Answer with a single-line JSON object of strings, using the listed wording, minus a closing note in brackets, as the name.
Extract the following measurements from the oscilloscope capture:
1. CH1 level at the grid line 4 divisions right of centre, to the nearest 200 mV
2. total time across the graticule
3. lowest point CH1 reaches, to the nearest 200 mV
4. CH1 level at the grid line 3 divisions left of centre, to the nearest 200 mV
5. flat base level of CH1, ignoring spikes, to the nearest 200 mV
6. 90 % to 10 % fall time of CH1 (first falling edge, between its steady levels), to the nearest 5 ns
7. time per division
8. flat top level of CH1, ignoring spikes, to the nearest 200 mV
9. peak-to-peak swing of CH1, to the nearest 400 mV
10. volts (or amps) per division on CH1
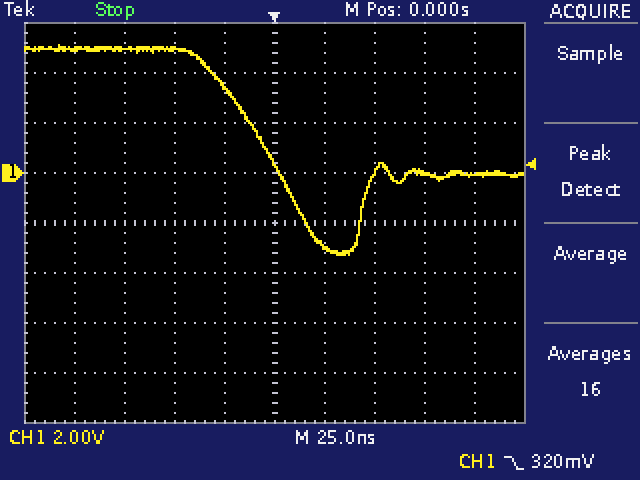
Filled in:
{"CH1 level at the grid line 4 divisions right of centre, to the nearest 200 mV": "0.0 V", "total time across the graticule": "250 ns", "lowest point CH1 reaches, to the nearest 200 mV": "-3.2 V", "CH1 level at the grid line 3 divisions left of centre, to the nearest 200 mV": "5.0 V", "flat base level of CH1, ignoring spikes, to the nearest 200 mV": "0.0 V", "90 % to 10 % fall time of CH1 (first falling edge, between its steady levels), to the nearest 5 ns": "35 ns", "time per division": "25 ns", "flat top level of CH1, ignoring spikes, to the nearest 200 mV": "5.0 V", "peak-to-peak swing of CH1, to the nearest 400 mV": "8.4 V", "volts (or amps) per division on CH1": "2 V"}
